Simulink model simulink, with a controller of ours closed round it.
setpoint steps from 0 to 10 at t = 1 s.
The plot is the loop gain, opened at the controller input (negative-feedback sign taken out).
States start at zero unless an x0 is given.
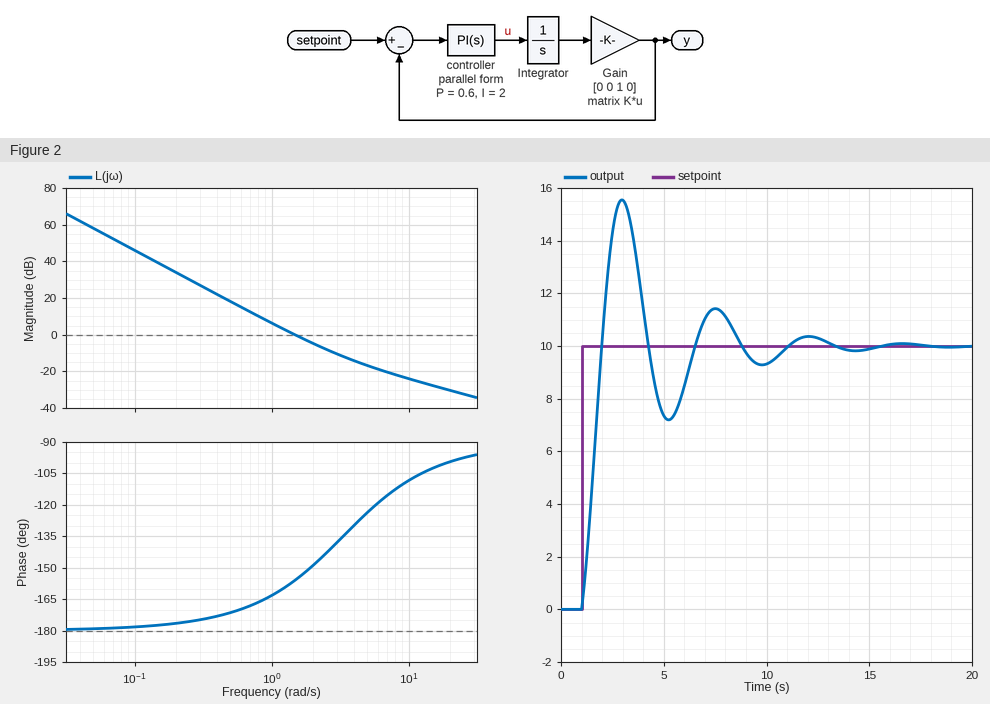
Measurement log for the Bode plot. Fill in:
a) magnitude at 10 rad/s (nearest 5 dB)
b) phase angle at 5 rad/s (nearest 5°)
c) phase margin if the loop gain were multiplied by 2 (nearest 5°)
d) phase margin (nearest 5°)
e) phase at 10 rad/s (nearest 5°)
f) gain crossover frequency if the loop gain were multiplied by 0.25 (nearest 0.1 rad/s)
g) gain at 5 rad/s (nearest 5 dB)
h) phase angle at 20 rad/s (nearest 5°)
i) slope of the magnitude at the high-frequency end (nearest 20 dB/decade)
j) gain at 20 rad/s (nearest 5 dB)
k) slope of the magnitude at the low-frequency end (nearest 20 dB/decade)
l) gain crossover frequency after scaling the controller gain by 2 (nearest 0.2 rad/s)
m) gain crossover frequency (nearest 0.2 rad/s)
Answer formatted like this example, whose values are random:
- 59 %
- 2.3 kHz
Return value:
- -25 dB
- -125°
- 35°
- 25°
- -110°
- 0.7 rad/s
- -15 dB
- -100°
- -20 dB/decade
- -30 dB
- -40 dB/decade
- 2.2 rad/s
- 1.4 rad/s
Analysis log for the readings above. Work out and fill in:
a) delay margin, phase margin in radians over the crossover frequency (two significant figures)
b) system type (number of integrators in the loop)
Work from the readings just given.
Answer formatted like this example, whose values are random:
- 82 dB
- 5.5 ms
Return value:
- 0.31 s
- 2
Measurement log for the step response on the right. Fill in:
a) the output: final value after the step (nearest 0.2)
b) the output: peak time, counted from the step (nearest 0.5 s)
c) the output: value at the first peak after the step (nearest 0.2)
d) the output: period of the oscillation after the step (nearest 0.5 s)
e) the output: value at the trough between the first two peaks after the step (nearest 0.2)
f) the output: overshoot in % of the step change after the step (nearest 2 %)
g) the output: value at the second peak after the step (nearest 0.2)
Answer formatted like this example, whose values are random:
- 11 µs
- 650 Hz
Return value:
- 10.0
- 2.0 s
- 15.6
- 4.5 s
- 7.2
- 56 %
- 11.4
